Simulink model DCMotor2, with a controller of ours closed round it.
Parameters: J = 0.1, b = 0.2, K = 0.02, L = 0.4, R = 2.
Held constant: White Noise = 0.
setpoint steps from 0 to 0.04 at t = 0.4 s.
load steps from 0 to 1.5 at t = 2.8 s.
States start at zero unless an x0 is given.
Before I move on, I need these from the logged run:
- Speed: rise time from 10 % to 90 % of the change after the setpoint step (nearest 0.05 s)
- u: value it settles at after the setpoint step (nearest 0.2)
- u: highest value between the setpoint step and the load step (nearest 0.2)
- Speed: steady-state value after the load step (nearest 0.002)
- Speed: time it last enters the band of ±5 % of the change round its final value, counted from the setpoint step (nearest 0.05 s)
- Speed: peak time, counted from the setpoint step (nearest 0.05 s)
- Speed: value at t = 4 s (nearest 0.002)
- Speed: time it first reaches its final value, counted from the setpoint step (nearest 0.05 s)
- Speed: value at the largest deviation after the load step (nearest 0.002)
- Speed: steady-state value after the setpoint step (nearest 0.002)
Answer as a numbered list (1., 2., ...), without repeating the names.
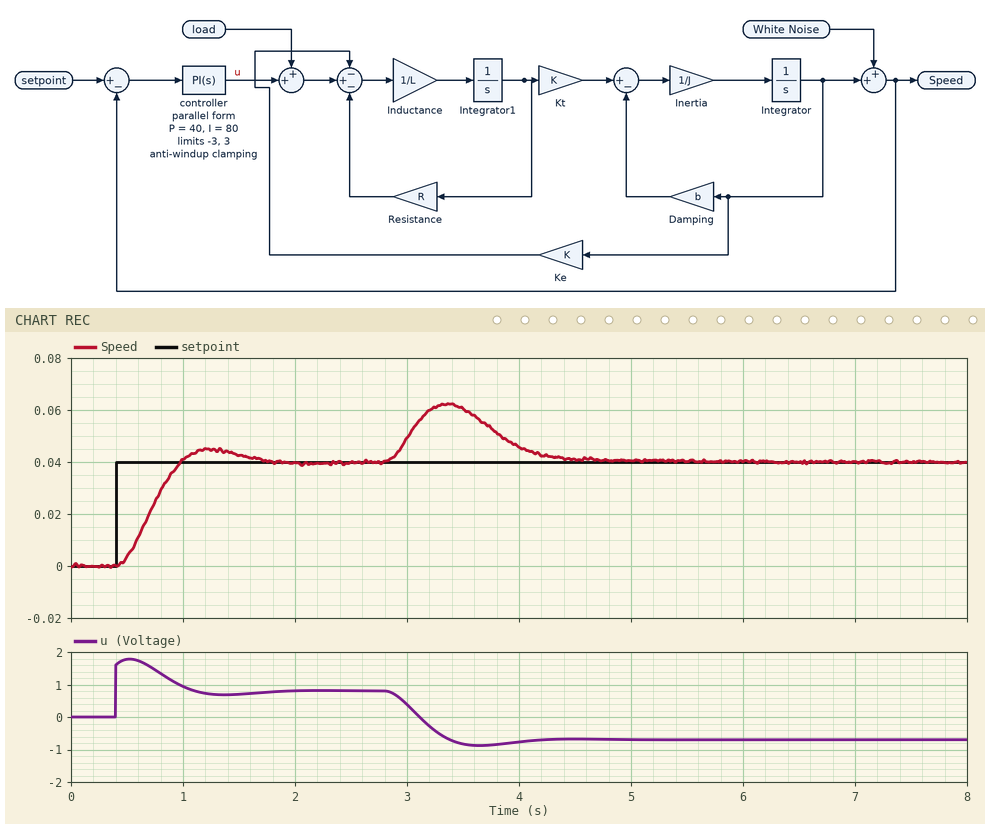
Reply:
1. 0.40 s
2. 0.8
3. 1.8
4. 0.040
5. 1.20 s
6. 0.85 s
7. 0.046
8. 0.60 s
9. 0.062
10. 0.040
